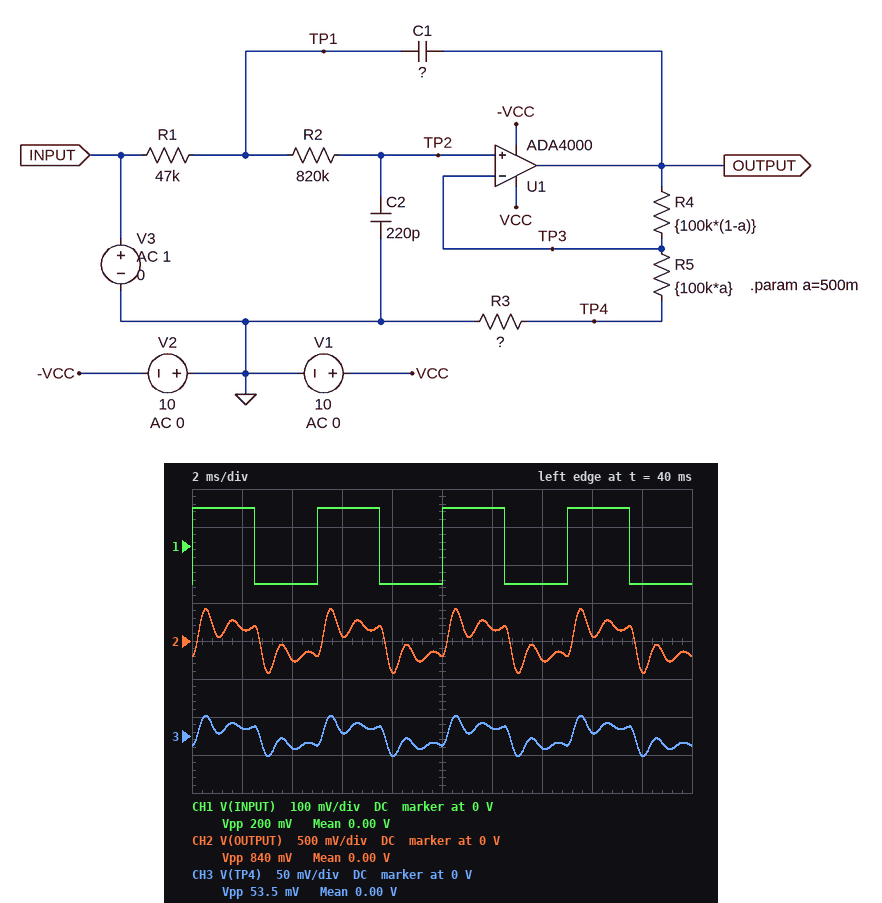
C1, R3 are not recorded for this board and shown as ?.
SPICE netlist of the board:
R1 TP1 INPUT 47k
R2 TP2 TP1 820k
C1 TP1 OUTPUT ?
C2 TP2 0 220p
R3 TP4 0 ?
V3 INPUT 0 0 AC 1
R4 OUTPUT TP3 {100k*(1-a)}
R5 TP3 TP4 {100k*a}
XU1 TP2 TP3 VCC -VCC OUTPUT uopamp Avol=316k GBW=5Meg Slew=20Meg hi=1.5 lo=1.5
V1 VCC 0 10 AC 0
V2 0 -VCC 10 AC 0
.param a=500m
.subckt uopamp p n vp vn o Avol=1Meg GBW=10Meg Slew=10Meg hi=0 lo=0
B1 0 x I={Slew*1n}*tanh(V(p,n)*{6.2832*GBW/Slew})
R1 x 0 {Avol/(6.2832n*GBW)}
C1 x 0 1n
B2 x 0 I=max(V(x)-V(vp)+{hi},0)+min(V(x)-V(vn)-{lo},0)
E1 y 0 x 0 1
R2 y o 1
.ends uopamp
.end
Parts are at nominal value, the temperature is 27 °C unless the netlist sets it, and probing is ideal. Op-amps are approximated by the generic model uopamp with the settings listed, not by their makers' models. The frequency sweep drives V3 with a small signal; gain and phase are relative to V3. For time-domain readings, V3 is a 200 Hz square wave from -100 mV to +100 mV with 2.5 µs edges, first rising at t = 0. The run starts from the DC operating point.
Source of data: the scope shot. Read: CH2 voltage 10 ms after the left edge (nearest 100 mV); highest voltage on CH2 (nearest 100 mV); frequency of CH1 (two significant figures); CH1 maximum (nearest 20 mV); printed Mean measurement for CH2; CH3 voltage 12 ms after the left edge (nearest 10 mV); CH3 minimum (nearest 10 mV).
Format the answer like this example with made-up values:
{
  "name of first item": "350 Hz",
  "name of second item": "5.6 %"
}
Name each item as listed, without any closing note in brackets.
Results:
{
  "CH2 voltage 10 ms after the left edge": "-200 mV",
  "highest voltage on CH2": "400 mV",
  "frequency of CH1": "200 Hz",
  "CH1 maximum": "100 mV",
  "printed Mean measurement for CH2": "0.00 V",
  "CH3 voltage 12 ms after the left edge": "10 mV",
  "CH3 minimum": "-30 mV"
}
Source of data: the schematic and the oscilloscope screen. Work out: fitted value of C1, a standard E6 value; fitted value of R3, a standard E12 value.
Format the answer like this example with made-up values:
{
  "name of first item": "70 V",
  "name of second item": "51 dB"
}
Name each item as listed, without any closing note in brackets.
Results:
{
  "fitted value of C1, a standard E6 value": "3.3 nF",
  "fitted value of R3, a standard E12 value": "6.8 kΩ"
}
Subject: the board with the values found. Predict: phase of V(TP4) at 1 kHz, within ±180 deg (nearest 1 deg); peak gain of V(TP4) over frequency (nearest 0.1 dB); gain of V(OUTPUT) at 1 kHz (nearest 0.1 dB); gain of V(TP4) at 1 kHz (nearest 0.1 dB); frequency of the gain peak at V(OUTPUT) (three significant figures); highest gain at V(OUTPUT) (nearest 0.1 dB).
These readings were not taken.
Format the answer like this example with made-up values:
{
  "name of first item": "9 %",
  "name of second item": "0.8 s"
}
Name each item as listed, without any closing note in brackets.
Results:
{
  "phase of V(TP4) at 1 kHz, within ±180 deg": "-107 deg",
  "peak gain of V(TP4) over frequency": "-8.5 dB",
  "gain of V(OUTPUT) at 1 kHz": "14.4 dB",
  "gain of V(TP4) at 1 kHz": "-9.5 dB",
  "frequency of the gain peak at V(OUTPUT)": "926 Hz",
  "highest gain at V(OUTPUT)": "15.4 dB"
}
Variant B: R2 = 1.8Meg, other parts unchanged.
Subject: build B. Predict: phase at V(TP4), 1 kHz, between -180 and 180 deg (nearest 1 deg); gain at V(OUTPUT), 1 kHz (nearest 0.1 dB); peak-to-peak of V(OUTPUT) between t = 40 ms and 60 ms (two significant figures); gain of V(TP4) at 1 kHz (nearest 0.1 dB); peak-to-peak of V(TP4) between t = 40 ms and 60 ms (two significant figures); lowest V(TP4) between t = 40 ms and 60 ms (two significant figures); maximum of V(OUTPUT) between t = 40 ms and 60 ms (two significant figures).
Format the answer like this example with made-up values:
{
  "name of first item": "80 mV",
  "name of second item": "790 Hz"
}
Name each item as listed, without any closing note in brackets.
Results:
{
  "phase at V(TP4), 1 kHz, between -180 and 180 deg": "-130 deg",
  "gain at V(OUTPUT), 1 kHz": "-1.4 dB",
  "peak-to-peak of V(OUTPUT) between t = 40 ms and 60 ms": "470 mV",
  "gain of V(TP4) at 1 kHz": "-25.3 dB",
  "peak-to-peak of V(TP4) between t = 40 ms and 60 ms": "30 mV",
  "lowest V(TP4) between t = 40 ms and 60 ms": "-15 mV",
  "maximum of V(OUTPUT) between t = 40 ms and 60 ms": "240 mV"
}
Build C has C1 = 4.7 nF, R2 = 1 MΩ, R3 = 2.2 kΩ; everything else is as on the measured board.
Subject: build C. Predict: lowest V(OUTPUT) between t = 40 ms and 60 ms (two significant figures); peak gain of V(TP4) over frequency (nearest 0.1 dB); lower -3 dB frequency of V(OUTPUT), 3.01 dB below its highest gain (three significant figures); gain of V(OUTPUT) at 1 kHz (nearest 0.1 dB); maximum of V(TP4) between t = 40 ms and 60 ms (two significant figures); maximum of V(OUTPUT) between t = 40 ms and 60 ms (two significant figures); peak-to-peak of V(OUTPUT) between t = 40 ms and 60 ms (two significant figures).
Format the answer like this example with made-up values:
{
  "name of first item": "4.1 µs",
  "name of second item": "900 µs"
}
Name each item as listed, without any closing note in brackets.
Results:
{
  "lowest V(OUTPUT) between t = 40 ms and 60 ms": "-460 mV",
  "peak gain of V(TP4) over frequency": "-6.1 dB",
  "lower -3 dB frequency of V(OUTPUT), 3.01 dB below its highest gain": "689 Hz",
  "gain of V(OUTPUT) at 1 kHz": "6.5 dB",
  "maximum of V(TP4) between t = 40 ms and 60 ms": "9.9 mV",
  "maximum of V(OUTPUT) between t = 40 ms and 60 ms": "460 mV",
  "peak-to-peak of V(OUTPUT) between t = 40 ms and 60 ms": "920 mV"
}
